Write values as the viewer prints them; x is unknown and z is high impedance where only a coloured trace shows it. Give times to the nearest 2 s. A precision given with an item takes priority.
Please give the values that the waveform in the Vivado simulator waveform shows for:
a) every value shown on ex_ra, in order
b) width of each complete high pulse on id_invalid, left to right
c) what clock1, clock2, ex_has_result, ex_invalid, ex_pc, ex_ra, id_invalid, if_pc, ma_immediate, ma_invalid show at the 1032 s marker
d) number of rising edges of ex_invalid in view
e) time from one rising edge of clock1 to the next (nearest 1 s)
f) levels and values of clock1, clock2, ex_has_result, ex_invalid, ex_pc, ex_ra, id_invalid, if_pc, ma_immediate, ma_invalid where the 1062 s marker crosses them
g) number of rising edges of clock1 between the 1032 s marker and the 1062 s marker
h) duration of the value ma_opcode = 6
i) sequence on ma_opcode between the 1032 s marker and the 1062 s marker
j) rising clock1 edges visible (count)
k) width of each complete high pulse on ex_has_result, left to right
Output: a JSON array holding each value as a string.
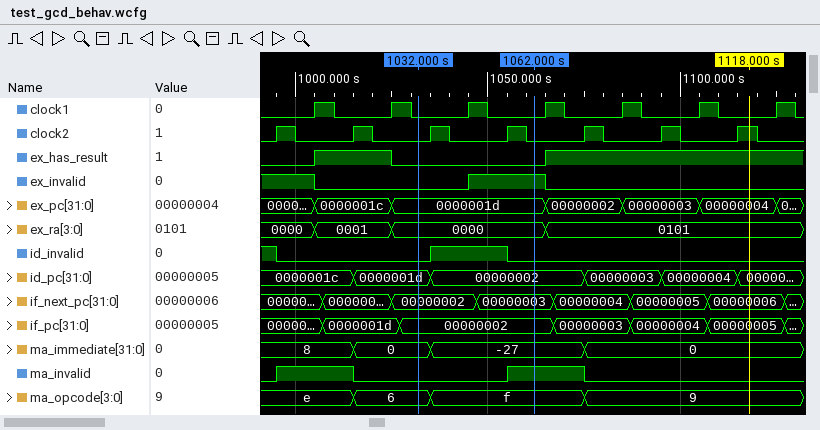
["0000, 0001, 0000, 0101", "20 s", "clock1=0, clock2=0, ex_has_result=0, ex_invalid=0, ex_pc=0000001d, ex_ra=0000, id_invalid=0, if_pc=00000002, ma_immediate=0, ma_invalid=0", "1", "20 s", "clock1=0, clock2=0, ex_has_result=0, ex_invalid=1, ex_pc=0000001d, ex_ra=0000, id_invalid=0, if_pc=00000002, ma_immediate=-27, ma_invalid=1", "1", "20 s", "6, f", "7", "20 s"]
